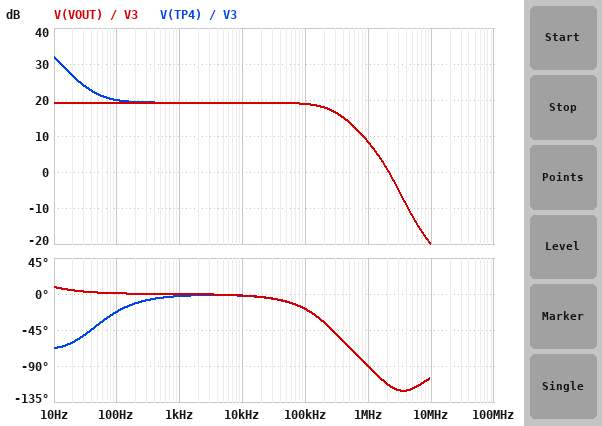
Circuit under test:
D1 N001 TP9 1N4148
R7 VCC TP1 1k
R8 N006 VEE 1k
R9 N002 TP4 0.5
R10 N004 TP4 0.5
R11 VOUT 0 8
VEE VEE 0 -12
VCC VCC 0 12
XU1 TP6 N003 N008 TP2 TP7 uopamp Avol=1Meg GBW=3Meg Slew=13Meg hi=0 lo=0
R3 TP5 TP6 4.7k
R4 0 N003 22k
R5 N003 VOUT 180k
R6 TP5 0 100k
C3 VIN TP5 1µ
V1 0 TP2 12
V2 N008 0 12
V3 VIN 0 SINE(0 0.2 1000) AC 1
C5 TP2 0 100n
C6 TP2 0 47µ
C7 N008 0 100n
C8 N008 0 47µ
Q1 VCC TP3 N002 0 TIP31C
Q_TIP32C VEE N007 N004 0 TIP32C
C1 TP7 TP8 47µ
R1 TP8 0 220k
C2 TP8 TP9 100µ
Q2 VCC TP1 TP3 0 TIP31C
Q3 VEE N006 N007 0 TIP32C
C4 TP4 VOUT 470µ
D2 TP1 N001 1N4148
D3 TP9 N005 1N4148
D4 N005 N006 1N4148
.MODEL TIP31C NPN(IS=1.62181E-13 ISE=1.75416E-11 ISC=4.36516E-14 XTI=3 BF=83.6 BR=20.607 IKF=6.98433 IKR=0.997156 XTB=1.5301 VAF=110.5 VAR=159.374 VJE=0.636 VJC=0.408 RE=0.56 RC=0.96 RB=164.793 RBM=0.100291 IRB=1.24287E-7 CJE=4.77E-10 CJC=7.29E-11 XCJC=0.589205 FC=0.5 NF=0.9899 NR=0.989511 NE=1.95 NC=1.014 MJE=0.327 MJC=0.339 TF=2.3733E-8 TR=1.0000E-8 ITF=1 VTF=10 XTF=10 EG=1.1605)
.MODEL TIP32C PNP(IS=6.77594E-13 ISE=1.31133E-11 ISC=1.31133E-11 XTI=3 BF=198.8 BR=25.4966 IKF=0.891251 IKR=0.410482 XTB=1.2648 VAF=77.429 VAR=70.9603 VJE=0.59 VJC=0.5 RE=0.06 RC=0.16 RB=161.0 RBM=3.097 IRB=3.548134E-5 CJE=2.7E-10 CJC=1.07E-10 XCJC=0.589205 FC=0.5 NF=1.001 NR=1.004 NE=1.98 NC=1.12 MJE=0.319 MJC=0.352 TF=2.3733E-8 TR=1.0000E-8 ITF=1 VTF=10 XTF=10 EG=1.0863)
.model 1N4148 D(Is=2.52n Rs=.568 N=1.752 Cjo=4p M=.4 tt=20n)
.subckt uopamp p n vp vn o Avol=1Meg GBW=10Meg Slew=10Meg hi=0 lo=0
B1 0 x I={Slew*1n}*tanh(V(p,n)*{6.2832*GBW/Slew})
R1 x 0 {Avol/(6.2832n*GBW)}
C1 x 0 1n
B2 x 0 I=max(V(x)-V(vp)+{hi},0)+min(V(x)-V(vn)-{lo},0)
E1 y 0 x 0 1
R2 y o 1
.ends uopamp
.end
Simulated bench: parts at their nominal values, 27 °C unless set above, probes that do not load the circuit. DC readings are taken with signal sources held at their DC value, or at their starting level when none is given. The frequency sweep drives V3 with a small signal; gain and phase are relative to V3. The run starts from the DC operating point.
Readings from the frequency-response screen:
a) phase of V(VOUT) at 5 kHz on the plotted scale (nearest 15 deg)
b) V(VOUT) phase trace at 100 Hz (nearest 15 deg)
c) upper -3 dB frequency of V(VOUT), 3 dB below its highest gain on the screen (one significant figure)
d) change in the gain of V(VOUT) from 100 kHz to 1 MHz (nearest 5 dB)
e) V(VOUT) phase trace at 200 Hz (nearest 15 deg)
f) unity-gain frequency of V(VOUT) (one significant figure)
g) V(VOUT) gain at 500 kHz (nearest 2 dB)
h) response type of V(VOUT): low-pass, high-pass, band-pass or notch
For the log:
0 deg
0 deg
300 kHz
-10 dB
0 deg
2 MHz
14 dB
low-pass
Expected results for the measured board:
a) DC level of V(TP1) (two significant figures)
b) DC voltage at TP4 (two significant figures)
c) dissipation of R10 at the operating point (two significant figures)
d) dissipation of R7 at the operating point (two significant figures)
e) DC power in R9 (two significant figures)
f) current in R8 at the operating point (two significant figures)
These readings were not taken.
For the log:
1.4 V
-77 mV
12 mW
110 mW
12 mW
11 mA
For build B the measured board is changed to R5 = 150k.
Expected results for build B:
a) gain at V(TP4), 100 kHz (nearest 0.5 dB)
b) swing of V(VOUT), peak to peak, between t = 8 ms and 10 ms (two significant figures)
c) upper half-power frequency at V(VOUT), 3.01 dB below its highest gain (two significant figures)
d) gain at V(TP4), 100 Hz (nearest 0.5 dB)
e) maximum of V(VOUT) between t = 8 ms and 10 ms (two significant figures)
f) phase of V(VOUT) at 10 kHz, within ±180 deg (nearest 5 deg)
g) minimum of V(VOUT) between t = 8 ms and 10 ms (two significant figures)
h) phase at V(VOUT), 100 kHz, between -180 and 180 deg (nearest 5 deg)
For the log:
17.5 dB
3.1 V
380 kHz
18.5 dB
1.6 V
0 deg
-1.6 V
-15 deg
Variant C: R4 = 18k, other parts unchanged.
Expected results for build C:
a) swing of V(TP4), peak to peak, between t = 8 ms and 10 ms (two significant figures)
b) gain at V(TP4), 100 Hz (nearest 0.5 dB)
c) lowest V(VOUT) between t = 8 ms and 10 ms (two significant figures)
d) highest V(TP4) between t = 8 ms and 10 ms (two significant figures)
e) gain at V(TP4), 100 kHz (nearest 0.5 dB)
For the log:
4.4 V
21.5 dB
-2.2 V
2.2 V
20.5 dB
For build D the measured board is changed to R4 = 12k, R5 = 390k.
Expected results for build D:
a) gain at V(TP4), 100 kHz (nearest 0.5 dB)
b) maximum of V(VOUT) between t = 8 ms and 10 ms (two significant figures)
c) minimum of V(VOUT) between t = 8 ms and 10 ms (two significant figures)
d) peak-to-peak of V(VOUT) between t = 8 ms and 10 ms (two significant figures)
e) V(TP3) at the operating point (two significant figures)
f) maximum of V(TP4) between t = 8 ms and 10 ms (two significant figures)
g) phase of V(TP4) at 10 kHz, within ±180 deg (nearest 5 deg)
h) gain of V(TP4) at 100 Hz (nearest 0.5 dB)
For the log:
26.5 dB
6.7 V
-6.7 V
13 V
800 mV
6.9 V
-5 deg
31.0 dB
